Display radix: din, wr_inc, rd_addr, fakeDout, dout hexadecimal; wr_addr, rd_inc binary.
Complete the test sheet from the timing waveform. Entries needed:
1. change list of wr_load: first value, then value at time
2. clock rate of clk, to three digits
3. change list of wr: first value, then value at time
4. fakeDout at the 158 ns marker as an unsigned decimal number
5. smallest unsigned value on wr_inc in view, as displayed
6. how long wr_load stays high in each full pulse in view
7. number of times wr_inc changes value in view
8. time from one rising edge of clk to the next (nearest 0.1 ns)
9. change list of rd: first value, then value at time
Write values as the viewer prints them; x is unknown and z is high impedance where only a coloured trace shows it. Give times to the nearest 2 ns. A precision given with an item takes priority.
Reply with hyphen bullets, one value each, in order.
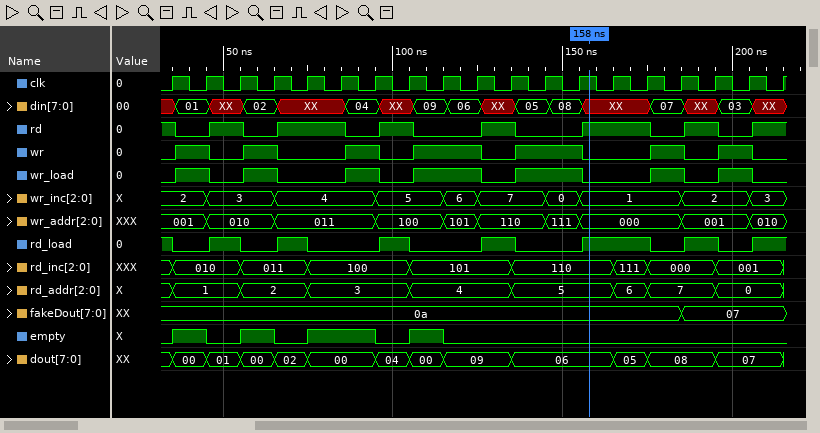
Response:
- 0, 1 at 36 ns, 0 at 46 ns, 1 at 56 ns, 0 at 66 ns, 1 at 86 ns, 0 at 96 ns, 1 at 106 ns, 0 at 126 ns, 1 at 136 ns, 0 at 156 ns, 1 at 176 ns, 0 at 186 ns, 1 at 196 ns, 0 at 206 ns
- 100 MHz
- 0, 1 at 36 ns, 0 at 46 ns, 1 at 56 ns, 0 at 66 ns, 1 at 86 ns, 0 at 96 ns, 1 at 106 ns, 0 at 126 ns, 1 at 136 ns, 0 at 156 ns, 1 at 176 ns, 0 at 186 ns, 1 at 196 ns, 0 at 206 ns
- 10
- 0
- 10 ns, 10 ns, 10 ns, 20 ns, 20 ns, 10 ns, 10 ns
- 9
- 10 ns
- 1, 0 at 36 ns, 1 at 46 ns, 0 at 56 ns, 1 at 66 ns, 0 at 86 ns, 1 at 96 ns, 0 at 106 ns, 1 at 126 ns, 0 at 136 ns, 1 at 156 ns, 0 at 176 ns, 1 at 186 ns, 0 at 196 ns, 1 at 206 ns
